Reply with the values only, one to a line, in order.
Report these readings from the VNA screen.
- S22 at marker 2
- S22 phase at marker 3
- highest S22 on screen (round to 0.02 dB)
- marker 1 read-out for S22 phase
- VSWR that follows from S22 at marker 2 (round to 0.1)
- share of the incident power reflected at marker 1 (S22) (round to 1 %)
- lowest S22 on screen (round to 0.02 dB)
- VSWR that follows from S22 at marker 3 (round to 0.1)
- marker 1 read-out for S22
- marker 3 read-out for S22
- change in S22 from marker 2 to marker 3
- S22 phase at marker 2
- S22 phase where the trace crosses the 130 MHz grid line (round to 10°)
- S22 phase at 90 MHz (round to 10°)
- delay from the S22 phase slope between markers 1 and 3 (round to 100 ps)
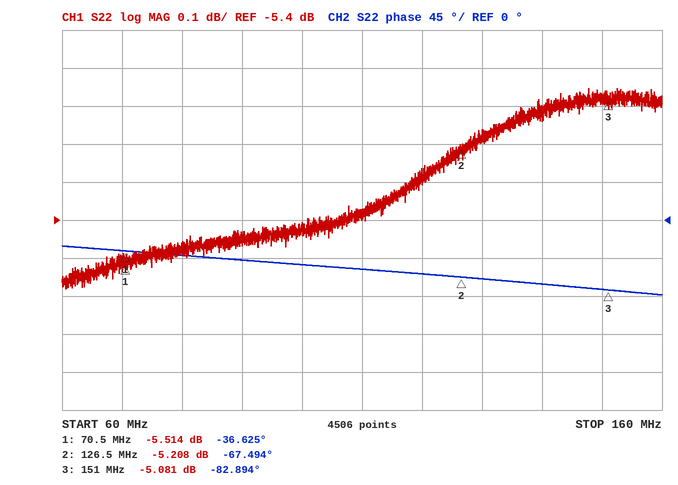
-5.208 dB
-82.894°
-5.06 dB
-36.625°
3.4
28 %
-5.58 dB
3.5
-5.514 dB
-5.081 dB
0.127 dB
-67.494°
-70°
-50°
1.6 ns
